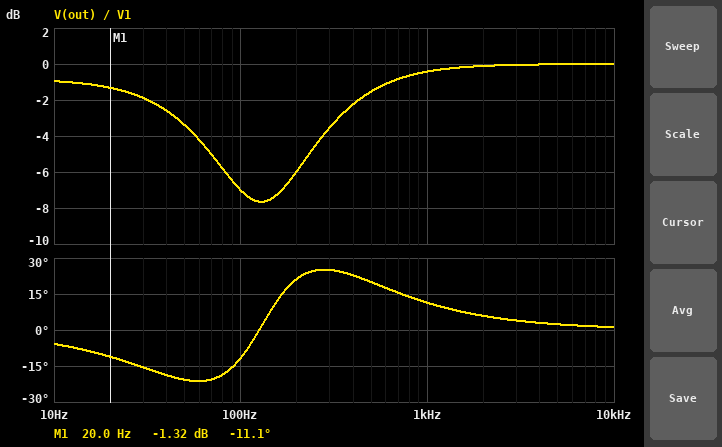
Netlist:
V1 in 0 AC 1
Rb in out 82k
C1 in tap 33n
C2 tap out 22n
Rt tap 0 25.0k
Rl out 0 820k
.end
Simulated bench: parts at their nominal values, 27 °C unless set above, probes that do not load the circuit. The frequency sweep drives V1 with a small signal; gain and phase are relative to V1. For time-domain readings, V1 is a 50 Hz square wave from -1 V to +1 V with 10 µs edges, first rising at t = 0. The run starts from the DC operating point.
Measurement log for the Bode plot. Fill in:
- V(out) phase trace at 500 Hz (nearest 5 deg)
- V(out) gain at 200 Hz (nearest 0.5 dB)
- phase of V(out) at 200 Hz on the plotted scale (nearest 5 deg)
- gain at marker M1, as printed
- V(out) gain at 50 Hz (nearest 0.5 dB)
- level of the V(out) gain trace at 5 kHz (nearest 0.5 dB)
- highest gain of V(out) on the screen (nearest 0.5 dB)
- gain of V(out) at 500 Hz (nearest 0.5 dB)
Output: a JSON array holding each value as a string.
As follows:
["20 deg", "-6.0 dB", "20 deg", "-1.32 dB", "-3.5 dB", "0 dB", "0 dB", "-1.5 dB"]
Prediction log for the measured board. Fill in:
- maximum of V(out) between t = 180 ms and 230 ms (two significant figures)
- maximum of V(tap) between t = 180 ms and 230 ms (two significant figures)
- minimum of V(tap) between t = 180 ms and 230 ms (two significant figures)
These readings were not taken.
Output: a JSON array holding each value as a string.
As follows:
["1.1 V", "2.0 V", "-2.0 V"]
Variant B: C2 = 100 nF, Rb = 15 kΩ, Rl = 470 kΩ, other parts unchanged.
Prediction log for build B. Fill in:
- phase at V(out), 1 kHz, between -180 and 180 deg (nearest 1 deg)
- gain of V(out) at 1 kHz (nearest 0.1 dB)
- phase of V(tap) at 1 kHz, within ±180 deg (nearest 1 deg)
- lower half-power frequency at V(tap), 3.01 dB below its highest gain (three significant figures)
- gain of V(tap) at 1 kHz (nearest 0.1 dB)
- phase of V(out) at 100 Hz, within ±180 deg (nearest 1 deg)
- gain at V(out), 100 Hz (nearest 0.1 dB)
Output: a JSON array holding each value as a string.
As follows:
["9 deg", "-0.8 dB", "10 deg", "127 Hz", "-0.6 dB", "-4 deg", "-3.3 dB"]
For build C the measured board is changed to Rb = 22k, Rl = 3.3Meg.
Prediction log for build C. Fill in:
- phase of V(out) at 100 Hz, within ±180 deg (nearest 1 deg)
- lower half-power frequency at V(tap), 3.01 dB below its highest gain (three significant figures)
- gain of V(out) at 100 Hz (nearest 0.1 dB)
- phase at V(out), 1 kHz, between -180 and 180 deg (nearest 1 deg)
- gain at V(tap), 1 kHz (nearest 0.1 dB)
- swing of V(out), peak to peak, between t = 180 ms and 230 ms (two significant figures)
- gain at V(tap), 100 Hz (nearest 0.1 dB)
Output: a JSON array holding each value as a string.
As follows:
["-8 deg", "143 Hz", "-1.6 dB", "8 deg", "-0.4 dB", "2.0 V", "-4.3 dB"]
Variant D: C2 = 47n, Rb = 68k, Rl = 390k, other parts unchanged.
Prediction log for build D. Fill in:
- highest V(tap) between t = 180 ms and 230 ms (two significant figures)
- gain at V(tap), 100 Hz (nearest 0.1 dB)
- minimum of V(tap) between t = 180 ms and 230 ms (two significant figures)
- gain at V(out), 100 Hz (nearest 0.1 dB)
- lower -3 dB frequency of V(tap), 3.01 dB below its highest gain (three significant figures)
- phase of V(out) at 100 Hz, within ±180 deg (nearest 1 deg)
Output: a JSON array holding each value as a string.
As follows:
["1.9 V", "-6.2 dB", "-1.9 V", "-8.9 dB", "241 Hz", "4 deg"]
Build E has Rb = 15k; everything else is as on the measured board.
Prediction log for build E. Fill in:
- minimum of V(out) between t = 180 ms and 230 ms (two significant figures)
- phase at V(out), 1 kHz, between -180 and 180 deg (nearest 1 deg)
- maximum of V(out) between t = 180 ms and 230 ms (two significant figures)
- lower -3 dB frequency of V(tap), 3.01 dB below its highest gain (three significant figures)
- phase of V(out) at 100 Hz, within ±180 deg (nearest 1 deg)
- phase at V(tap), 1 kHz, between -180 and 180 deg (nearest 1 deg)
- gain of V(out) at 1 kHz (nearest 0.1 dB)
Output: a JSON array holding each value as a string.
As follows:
["-1.0 V", "7 deg", "1.0 V", "133 Hz", "-6 deg", "9 deg", "-1.0 dB"]
